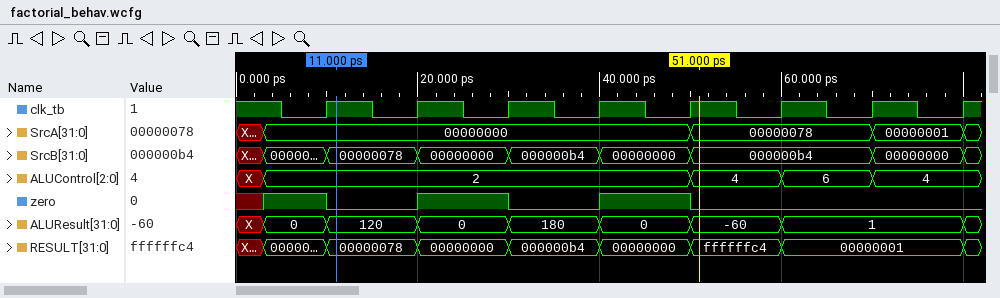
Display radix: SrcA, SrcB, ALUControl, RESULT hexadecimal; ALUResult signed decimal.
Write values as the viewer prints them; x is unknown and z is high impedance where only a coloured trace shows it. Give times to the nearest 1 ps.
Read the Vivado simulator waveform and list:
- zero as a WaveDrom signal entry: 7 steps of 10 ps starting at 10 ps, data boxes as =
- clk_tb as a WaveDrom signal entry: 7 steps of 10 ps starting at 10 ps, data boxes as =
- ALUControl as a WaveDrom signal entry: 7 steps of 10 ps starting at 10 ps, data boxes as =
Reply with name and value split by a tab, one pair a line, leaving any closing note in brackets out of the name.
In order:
zero as a WaveDrom signal entry: 7 steps of 10 ps starting at 10 ps, data boxes as =	{name: 'zero', wave: '01010..'}
clk_tb as a WaveDrom signal entry: 7 steps of 10 ps starting at 10 ps, data boxes as =	{name: 'clk_tb', wave: 'p......'}
ALUControl as a WaveDrom signal entry: 7 steps of 10 ps starting at 10 ps, data boxes as =	{name: 'ALUControl', wave: '=...===', data: '2 4 6 4'}
